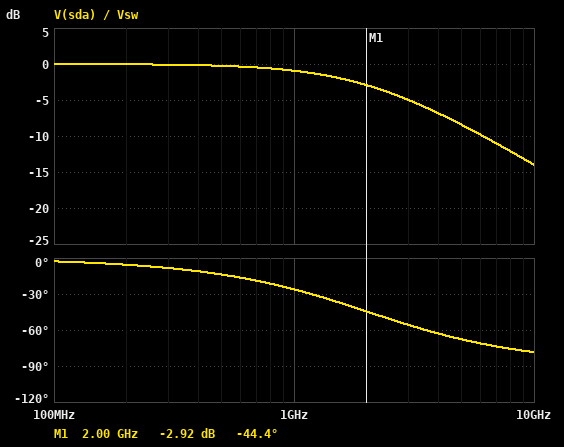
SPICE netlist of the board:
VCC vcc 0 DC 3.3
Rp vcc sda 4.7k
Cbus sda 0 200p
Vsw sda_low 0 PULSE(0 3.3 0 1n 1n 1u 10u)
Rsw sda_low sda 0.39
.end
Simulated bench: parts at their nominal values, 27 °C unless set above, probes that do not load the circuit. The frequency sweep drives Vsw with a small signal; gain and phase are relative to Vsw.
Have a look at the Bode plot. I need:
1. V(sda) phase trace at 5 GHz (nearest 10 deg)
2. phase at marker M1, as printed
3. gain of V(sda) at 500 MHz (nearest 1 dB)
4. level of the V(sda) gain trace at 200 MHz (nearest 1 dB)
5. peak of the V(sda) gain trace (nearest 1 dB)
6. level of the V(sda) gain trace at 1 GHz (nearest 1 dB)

-70 deg
-44.4 deg
0 dB
0 dB
0 dB
-1 dB
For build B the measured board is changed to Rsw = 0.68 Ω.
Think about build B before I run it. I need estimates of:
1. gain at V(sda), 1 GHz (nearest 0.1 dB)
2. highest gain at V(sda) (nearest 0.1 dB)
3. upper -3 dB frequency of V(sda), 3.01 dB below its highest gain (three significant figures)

-2.4 dB
0 dB
1.17 GHz
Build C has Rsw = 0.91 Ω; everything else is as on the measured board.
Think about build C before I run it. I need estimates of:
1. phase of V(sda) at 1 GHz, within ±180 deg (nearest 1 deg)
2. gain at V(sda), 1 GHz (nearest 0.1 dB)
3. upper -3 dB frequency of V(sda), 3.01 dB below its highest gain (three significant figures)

-49 deg
-3.6 dB
875 MHz
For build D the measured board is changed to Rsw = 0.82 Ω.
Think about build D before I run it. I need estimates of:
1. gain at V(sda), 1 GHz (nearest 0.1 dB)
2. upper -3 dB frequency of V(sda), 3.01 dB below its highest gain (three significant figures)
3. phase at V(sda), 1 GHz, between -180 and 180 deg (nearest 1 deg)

-3.1 dB
971 MHz
-46 deg
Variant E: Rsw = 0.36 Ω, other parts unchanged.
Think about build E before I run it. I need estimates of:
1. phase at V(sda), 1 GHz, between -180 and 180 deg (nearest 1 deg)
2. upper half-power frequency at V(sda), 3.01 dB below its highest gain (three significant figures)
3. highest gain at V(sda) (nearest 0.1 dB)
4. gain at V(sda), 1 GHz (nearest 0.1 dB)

-24 deg
2.21 GHz
0 dB
-0.8 dB
